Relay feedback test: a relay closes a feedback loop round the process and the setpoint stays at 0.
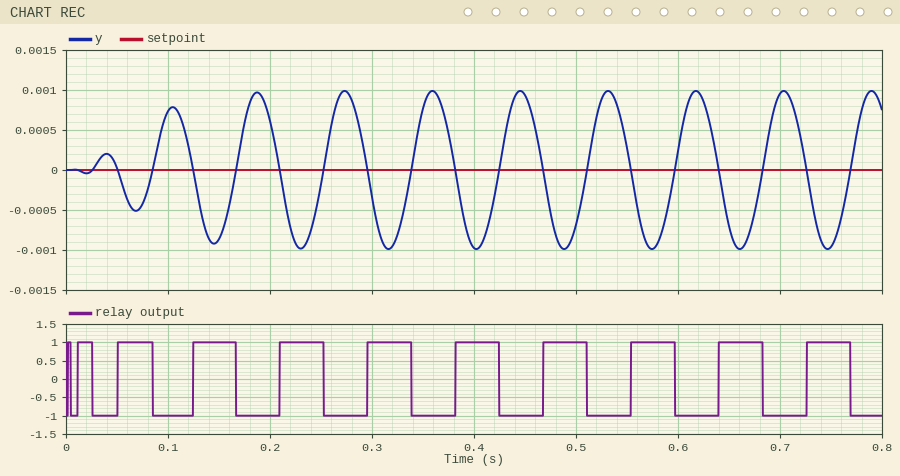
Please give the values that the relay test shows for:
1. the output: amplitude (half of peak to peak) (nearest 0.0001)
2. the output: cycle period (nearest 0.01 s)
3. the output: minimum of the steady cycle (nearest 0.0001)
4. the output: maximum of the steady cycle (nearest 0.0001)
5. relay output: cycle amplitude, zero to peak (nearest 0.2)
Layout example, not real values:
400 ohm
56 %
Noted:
0.0010
0.09 s
-0.0010
0.0010
1.0
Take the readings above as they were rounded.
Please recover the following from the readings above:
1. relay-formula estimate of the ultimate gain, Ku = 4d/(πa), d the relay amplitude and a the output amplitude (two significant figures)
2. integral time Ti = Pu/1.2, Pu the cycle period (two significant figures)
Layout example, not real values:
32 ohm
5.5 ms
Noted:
1300
0.075 s
